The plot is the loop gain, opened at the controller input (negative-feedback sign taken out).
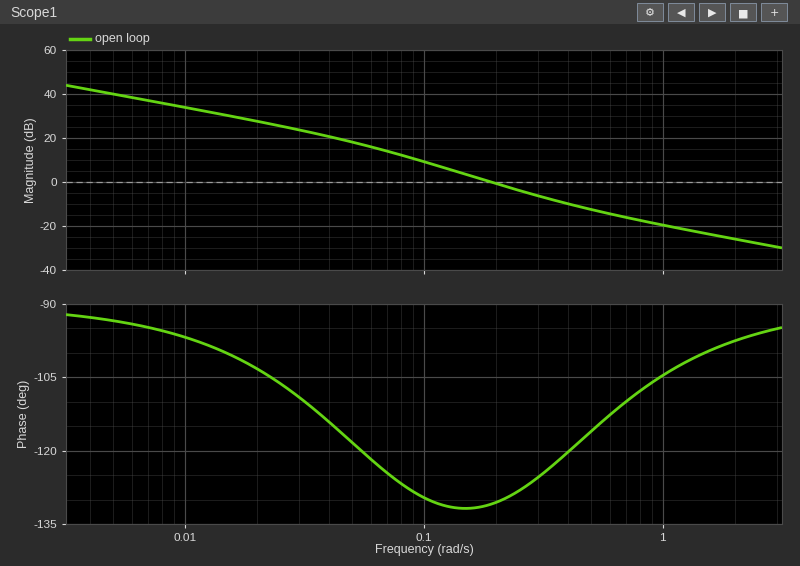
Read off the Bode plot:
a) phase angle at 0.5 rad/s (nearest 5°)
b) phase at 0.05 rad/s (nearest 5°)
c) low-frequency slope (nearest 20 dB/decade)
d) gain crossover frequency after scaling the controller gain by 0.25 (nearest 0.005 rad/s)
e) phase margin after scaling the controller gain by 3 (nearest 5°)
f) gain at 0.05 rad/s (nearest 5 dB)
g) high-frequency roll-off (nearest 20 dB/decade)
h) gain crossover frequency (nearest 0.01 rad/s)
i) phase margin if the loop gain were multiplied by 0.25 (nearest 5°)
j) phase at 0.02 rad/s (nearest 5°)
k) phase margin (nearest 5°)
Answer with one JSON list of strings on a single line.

["-115°", "-120°", "-20 dB/decade", "0.080 rad/s", "60°", "20 dB", "-20 dB/decade", "0.19 rad/s", "55°", "-105°", "50°"]
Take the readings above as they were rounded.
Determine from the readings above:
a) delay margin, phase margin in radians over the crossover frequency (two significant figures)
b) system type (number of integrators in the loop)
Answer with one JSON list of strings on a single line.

["4.6 s", "1"]
